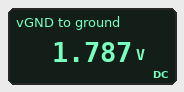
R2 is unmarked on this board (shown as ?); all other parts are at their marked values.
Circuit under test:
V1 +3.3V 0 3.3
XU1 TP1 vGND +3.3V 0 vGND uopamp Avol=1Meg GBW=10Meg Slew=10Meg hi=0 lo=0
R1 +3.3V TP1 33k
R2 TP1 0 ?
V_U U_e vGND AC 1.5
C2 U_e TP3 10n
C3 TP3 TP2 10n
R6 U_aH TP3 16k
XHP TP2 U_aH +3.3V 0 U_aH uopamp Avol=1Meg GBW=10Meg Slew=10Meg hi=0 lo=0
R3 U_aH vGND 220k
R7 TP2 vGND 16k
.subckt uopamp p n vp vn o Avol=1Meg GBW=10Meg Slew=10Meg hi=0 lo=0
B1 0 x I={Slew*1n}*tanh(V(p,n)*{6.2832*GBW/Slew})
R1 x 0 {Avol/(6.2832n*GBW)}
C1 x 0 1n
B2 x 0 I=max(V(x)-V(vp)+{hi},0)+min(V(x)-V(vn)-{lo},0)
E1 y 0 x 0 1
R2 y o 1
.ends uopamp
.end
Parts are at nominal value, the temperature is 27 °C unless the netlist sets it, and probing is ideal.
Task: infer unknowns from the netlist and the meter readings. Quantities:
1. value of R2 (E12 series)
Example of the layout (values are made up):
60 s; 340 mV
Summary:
39 kΩ
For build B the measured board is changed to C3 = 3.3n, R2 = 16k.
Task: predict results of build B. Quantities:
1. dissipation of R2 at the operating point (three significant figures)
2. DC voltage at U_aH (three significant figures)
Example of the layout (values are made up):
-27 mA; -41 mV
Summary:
72.6 µW; 1.08 V
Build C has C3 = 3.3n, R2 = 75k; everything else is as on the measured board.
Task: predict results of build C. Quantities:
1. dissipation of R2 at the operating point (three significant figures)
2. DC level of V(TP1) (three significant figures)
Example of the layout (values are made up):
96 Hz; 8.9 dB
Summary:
70.0 µW; 2.29 V
